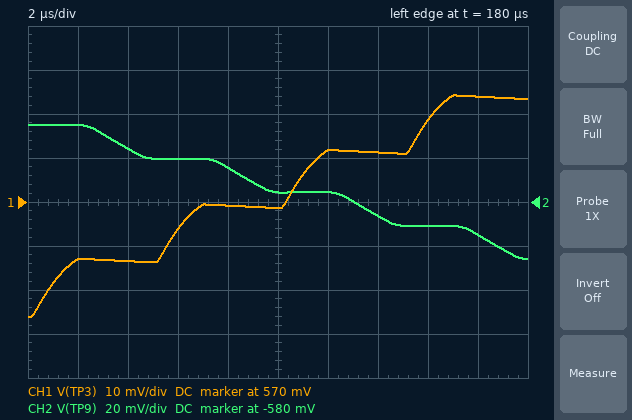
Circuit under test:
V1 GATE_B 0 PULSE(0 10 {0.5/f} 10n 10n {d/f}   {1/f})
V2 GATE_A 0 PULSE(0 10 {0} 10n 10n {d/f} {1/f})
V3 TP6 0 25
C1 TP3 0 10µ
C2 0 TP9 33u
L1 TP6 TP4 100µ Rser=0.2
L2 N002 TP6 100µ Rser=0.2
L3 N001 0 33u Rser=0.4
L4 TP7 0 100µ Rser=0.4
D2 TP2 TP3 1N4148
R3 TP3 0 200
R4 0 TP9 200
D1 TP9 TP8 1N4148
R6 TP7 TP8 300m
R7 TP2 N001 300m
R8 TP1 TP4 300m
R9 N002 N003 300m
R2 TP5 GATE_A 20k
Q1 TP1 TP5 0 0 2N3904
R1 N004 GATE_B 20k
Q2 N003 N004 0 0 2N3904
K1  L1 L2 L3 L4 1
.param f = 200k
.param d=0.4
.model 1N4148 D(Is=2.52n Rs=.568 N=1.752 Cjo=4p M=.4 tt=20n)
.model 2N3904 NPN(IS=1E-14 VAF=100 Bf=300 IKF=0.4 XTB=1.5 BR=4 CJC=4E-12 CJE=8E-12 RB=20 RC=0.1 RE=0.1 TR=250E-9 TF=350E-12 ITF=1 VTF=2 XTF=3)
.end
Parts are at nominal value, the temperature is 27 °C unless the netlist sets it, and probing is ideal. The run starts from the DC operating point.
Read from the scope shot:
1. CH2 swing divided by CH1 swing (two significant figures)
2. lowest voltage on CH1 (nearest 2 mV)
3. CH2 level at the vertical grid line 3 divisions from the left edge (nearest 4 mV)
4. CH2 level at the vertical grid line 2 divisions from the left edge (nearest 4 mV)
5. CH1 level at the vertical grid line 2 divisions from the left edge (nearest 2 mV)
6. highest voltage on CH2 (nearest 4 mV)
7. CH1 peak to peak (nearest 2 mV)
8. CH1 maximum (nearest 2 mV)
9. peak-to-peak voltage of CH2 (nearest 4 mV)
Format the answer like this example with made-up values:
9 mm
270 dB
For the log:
1.2
544 mV
-560 mV
-556 mV
556 mV
-544 mV
50 mV
594 mV
60 mV
